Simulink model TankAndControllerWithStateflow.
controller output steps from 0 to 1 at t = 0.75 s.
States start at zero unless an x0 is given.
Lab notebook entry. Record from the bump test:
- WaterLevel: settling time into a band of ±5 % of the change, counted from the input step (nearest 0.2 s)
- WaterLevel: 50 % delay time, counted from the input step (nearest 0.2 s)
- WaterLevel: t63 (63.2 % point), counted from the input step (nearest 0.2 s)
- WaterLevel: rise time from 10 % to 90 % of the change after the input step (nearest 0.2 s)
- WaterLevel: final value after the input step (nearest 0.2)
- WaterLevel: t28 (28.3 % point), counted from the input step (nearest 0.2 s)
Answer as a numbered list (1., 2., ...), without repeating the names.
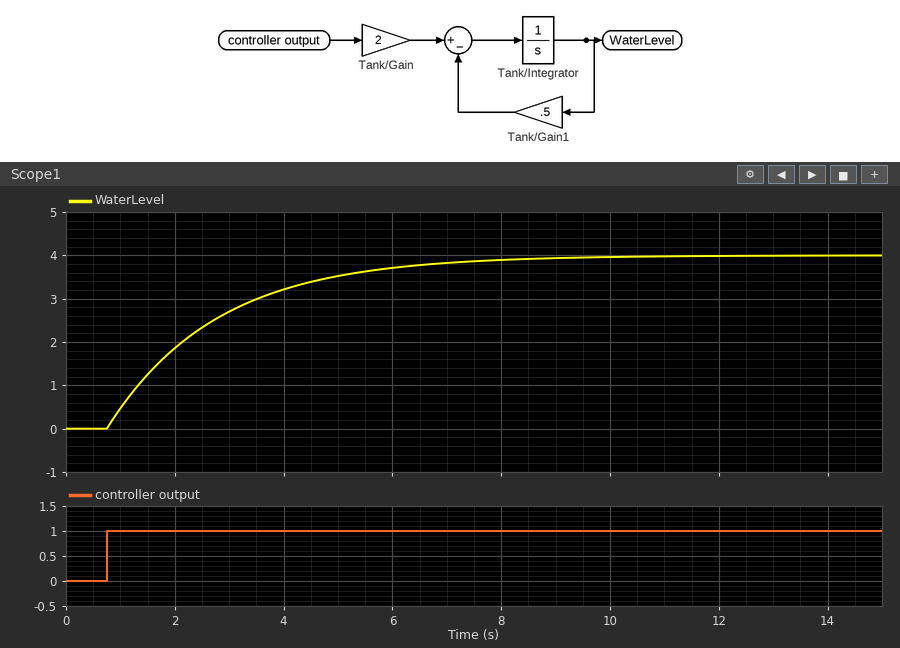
1. 6.0 s
2. 1.4 s
3. 2.0 s
4. 4.4 s
5. 4.0
6. 0.6 s
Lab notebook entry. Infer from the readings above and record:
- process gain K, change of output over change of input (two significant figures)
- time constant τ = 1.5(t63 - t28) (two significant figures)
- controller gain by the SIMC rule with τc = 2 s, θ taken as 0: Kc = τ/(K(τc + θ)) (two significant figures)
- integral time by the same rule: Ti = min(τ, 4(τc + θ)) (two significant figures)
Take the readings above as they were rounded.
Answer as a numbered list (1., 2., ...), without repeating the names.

1. 4.0
2. 2.1 s
3. 0.26
4. 2.1 s
